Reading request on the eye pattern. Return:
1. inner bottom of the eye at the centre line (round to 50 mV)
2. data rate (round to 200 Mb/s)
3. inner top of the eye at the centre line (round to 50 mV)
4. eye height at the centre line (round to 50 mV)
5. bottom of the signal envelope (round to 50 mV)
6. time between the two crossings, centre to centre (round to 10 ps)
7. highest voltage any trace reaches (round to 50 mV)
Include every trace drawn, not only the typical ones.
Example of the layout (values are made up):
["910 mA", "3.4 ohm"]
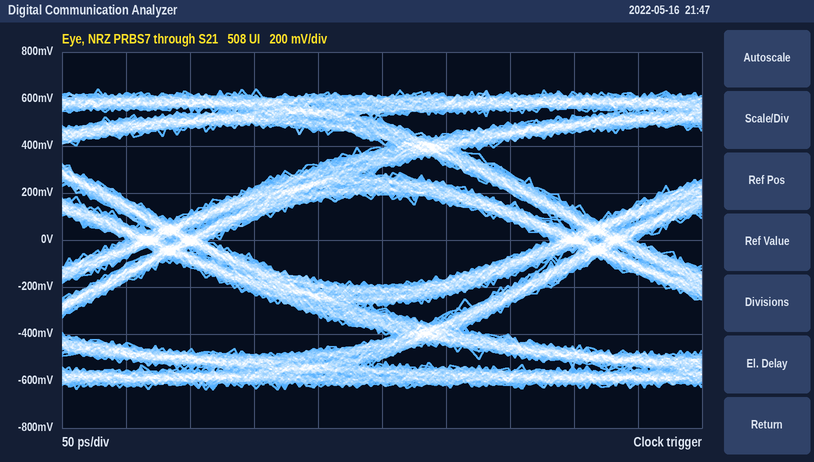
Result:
["-200 mV", "3.0 Gb/s", "200 mV", "400 mV", "-650 mV", "330 ps", "650 mV"]
